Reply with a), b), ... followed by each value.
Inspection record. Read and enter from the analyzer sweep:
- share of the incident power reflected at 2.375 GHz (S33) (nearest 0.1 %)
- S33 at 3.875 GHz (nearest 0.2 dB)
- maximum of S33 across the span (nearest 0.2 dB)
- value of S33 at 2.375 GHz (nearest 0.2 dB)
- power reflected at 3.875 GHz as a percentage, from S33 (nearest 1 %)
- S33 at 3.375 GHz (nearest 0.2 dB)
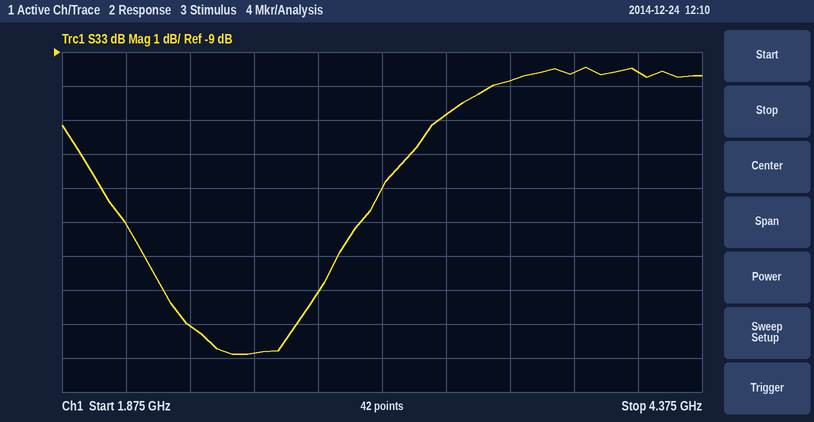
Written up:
a) 2.0 %
b) -9.6 dB
c) -9.4 dB
d) -17.0 dB
e) 11 %
f) -10.8 dB
